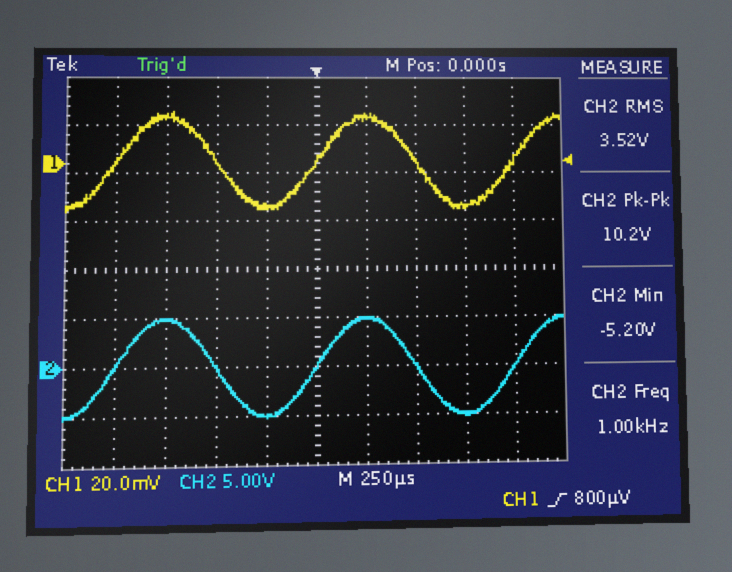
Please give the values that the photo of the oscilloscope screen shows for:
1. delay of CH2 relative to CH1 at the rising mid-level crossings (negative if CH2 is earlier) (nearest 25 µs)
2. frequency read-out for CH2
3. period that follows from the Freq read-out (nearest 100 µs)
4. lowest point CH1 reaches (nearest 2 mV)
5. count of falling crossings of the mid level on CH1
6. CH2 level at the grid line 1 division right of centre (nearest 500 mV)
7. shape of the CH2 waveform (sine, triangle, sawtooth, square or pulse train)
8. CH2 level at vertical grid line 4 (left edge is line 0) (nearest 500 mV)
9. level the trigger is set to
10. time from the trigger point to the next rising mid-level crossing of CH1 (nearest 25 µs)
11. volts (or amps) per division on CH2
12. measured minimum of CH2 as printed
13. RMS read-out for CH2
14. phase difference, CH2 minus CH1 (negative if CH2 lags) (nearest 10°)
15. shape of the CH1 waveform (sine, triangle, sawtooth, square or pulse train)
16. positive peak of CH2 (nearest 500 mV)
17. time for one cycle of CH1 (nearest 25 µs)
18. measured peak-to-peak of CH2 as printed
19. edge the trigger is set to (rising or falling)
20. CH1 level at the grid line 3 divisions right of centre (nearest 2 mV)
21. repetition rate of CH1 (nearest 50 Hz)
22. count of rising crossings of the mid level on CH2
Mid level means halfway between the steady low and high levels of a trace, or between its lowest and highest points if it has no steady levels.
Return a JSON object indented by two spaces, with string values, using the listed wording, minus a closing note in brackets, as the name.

{
  "delay of CH2 relative to CH1 at the rising mid-level crossings (negative if CH2 is earlier)": "0 µs",
  "frequency read-out for CH2": "1.00 kHz",
  "period that follows from the Freq read-out": "1.0 ms",
  "lowest point CH1 reaches": "-20 mV",
  "count of falling crossings of the mid level on CH1": "2",
  "CH2 level at the grid line 1 division right of centre": "5.0 V",
  "shape of the CH2 waveform": "sine",
  "CH2 level at vertical grid line 4 (left edge is line 0)": "-5.0 V",
  "level the trigger is set to": "800 µV",
  "time from the trigger point to the next rising mid-level crossing of CH1": "1.000 ms",
  "volts (or amps) per division on CH2": "5 V",
  "measured minimum of CH2 as printed": "-5.20 V",
  "RMS read-out for CH2": "3.52 V",
  "phase difference, CH2 minus CH1 (negative if CH2 lags)": "0°",
  "shape of the CH1 waveform": "sine",
  "positive peak of CH2": "5.0 V",
  "time for one cycle of CH1": "1.000 ms",
  "measured peak-to-peak of CH2 as printed": "10.2 V",
  "edge the trigger is set to": "rising",
  "CH1 level at the grid line 3 divisions right of centre": "-18 mV",
  "repetition rate of CH1": "1.00 kHz",
  "count of rising crossings of the mid level on CH2": "3"
}
